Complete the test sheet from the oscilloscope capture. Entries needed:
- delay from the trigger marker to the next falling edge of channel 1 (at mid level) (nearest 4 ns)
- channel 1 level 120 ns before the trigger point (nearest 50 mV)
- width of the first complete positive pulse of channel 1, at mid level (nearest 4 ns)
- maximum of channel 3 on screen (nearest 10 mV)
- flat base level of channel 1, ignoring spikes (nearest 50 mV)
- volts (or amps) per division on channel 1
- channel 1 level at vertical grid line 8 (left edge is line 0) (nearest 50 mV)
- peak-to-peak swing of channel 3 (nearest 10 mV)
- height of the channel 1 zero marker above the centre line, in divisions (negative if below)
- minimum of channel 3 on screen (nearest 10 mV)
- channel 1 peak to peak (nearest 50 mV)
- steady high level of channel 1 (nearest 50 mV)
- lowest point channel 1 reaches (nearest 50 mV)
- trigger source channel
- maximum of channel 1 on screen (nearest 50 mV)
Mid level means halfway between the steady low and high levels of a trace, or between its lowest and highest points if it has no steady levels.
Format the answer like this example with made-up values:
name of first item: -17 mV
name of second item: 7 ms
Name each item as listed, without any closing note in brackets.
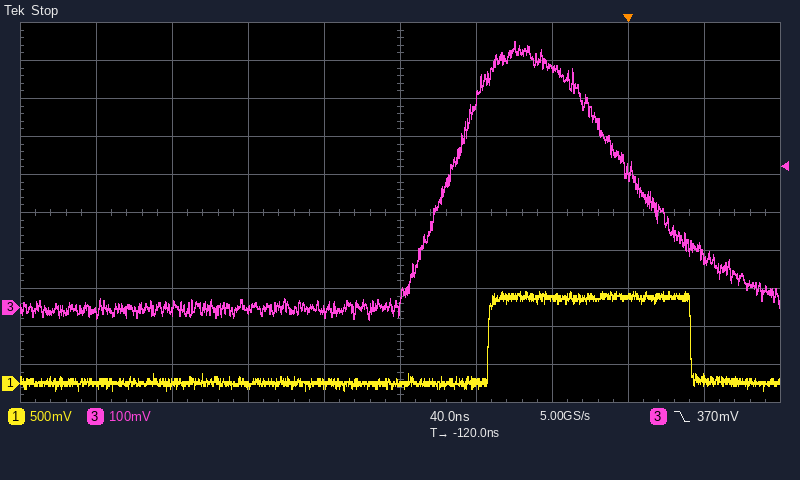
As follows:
delay from the trigger marker to the next falling edge of channel 1 (at mid level): 32 ns
channel 1 level 120 ns before the trigger point: 0 mV
width of the first complete positive pulse of channel 1, at mid level: 108 ns
maximum of channel 3 on screen: 700 mV
flat base level of channel 1, ignoring spikes: 0 mV
volts (or amps) per division on channel 1: 500 mV
channel 1 level at vertical grid line 8 (left edge is line 0): 1.15 V
peak-to-peak swing of channel 3: 730 mV
height of the channel 1 zero marker above the centre line, in divisions: -4.5 div
minimum of channel 3 on screen: -30 mV
channel 1 peak to peak: 1.30 V
steady high level of channel 1: 1.15 V
lowest point channel 1 reaches: -100 mV
trigger source channel: channel 3
maximum of channel 1 on screen: 1.20 V
